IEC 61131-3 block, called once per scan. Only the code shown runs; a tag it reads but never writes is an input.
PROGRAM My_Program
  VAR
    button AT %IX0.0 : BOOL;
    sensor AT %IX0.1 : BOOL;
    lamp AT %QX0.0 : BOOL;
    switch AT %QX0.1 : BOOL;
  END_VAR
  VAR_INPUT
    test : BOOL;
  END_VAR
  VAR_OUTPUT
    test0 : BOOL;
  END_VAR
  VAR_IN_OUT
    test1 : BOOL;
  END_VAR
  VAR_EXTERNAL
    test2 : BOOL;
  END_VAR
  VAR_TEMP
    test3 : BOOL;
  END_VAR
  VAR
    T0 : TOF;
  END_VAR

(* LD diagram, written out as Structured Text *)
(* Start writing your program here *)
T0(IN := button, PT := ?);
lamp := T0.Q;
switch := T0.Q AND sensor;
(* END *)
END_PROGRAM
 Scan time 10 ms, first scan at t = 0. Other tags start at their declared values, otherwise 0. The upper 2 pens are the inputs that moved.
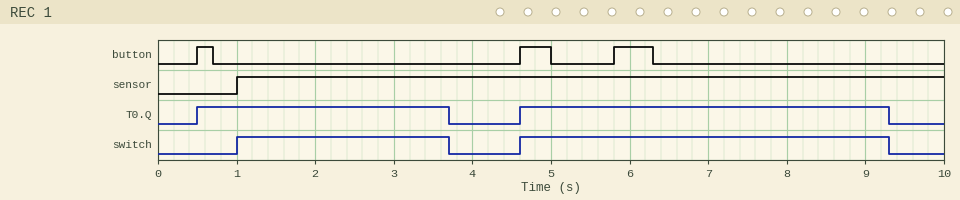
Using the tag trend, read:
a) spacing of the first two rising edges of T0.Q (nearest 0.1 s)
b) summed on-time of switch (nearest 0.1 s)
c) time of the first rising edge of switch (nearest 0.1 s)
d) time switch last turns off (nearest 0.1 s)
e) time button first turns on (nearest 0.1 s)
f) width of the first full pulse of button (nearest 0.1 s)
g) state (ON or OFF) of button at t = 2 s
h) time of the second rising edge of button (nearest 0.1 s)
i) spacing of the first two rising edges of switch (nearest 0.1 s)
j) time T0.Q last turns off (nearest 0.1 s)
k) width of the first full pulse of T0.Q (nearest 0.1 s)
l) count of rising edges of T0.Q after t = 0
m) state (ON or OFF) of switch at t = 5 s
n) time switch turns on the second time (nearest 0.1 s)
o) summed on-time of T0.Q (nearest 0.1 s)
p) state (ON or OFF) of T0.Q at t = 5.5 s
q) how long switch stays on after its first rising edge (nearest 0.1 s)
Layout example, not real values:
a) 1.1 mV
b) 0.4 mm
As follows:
a) 4.1 s
b) 7.4 s
c) 1.0 s
d) 9.3 s
e) 0.5 s
f) 0.2 s
g) OFF
h) 4.6 s
i) 3.6 s
j) 9.3 s
k) 3.2 s
l) 2
m) ON
n) 4.6 s
o) 7.9 s
p) ON
q) 2.7 s
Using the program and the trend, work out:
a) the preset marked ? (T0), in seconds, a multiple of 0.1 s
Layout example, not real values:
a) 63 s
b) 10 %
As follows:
a) 3.0 s
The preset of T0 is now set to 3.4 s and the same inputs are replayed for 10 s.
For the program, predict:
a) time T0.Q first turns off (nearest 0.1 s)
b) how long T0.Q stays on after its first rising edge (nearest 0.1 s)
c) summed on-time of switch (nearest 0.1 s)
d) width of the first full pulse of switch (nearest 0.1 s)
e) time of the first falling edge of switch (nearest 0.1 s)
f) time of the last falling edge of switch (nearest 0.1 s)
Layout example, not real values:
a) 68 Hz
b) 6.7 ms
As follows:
a) 4.1 s
b) 3.6 s
c) 8.2 s
d) 3.1 s
e) 4.1 s
f) 9.7 s
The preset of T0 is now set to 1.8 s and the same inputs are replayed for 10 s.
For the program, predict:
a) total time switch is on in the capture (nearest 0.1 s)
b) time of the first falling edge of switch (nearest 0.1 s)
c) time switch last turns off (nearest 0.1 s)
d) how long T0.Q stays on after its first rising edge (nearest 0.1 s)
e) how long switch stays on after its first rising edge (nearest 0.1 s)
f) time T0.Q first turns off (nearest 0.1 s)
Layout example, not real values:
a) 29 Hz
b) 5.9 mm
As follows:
a) 5.0 s
b) 2.5 s
c) 8.1 s
d) 2.0 s
e) 1.5 s
f) 2.5 s
